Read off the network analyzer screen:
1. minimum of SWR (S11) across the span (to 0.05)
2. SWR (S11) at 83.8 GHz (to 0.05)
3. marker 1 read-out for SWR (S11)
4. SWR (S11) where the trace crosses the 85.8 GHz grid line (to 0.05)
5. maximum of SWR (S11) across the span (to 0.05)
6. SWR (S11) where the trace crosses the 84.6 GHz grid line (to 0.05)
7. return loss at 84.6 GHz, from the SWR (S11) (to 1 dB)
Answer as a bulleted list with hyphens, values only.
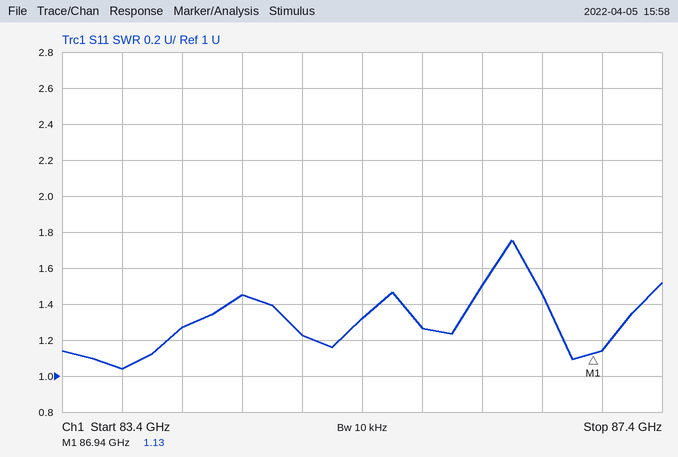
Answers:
- 1.05
- 1.05
- 1.13
- 1.25
- 1.75
- 1.45
- 15 dB
